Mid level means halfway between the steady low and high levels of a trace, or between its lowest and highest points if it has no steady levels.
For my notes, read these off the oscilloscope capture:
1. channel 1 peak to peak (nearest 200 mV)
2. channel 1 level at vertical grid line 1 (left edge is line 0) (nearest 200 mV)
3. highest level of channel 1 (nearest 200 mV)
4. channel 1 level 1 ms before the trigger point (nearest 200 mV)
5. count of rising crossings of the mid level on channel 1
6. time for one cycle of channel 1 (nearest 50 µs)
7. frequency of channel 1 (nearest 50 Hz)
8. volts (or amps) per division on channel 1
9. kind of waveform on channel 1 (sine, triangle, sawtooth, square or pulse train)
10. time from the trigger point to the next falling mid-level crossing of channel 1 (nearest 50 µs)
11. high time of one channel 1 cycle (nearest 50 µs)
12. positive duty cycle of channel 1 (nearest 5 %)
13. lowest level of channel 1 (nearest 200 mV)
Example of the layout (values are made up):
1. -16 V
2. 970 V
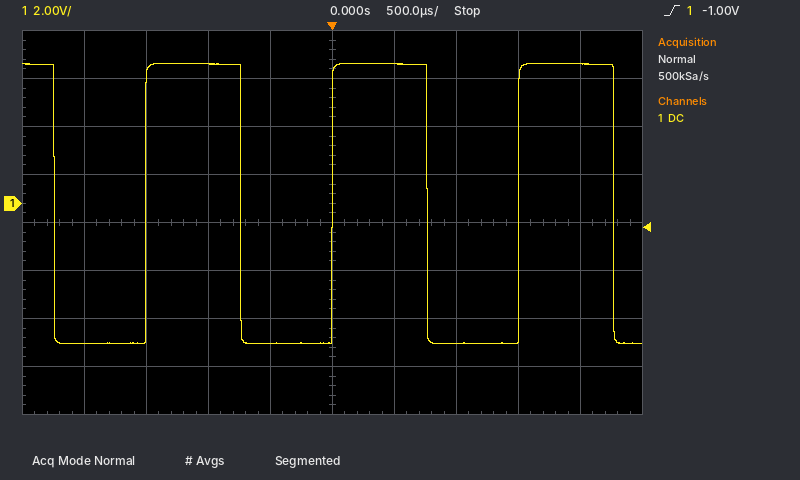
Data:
1. 11.6 V
2. -5.8 V
3. 5.8 V
4. 5.8 V
5. 3
6. 1.50 ms
7. 650 Hz
8. 2 V
9. square
10. 750 µs
11. 750 µs
12. 50 %
13. -5.8 V
